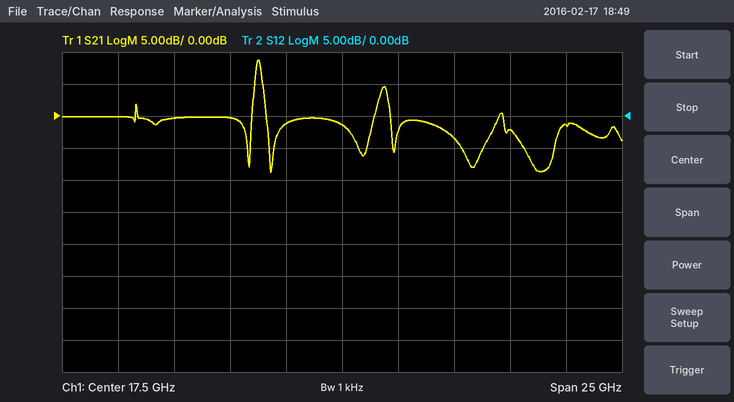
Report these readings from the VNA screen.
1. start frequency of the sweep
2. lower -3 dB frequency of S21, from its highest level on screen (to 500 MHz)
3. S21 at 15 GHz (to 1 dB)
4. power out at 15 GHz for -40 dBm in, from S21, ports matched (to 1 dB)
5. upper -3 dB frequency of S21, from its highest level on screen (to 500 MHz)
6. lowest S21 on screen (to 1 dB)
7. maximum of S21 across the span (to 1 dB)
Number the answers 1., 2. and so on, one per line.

1. 5 GHz
2. 13.5 GHz
3. -1 dB
4. -41 dBm
5. 14.0 GHz
6. -9 dB
7. 9 dB
